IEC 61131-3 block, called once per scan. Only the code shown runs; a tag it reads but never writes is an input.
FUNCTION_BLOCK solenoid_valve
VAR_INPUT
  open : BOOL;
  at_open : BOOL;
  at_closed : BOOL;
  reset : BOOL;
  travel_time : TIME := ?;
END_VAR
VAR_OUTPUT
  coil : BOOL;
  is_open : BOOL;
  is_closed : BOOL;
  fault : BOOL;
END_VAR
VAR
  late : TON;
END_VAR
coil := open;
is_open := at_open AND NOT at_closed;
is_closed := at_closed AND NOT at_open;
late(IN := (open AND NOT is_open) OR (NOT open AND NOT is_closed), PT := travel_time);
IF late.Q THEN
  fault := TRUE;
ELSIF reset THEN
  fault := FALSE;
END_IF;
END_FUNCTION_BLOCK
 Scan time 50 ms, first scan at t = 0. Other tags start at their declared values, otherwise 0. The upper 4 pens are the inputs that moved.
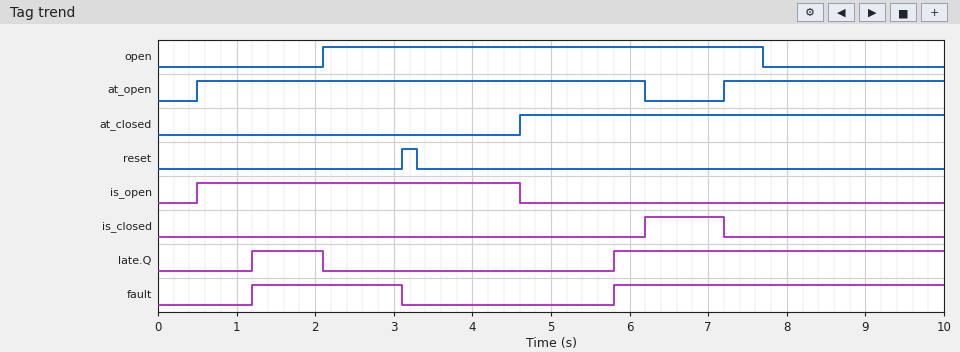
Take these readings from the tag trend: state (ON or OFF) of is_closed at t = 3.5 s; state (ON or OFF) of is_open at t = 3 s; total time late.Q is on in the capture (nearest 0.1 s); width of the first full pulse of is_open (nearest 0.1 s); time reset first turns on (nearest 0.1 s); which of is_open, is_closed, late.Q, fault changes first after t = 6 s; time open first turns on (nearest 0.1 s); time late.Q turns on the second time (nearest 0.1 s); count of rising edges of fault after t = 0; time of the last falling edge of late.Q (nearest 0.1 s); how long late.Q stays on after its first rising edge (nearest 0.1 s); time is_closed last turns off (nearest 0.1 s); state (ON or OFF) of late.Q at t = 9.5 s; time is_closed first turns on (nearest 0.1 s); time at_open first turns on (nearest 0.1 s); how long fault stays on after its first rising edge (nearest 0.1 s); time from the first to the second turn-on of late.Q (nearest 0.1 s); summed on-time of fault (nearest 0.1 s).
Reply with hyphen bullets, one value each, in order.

- OFF
- ON
- 5.1 s
- 4.1 s
- 3.1 s
- is_closed
- 2.1 s
- 5.8 s
- 2
- 2.1 s
- 0.9 s
- 7.2 s
- ON
- 6.2 s
- 0.5 s
- 1.9 s
- 4.6 s
- 6.1 s
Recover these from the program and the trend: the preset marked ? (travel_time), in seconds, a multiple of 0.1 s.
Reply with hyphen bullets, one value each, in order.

- 1.2 s
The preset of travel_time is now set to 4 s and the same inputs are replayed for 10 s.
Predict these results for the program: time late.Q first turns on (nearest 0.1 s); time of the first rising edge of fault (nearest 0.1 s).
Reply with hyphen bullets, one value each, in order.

- 8.6 s
- 8.6 s
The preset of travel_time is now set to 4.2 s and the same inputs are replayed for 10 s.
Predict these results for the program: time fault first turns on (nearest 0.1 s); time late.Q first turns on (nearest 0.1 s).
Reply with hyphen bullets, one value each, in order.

- 8.8 s
- 8.8 s
